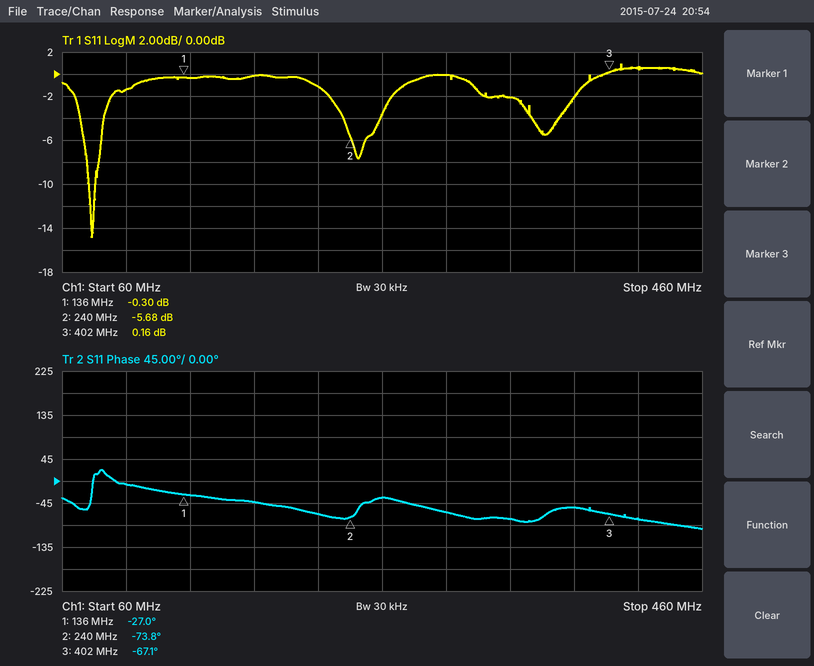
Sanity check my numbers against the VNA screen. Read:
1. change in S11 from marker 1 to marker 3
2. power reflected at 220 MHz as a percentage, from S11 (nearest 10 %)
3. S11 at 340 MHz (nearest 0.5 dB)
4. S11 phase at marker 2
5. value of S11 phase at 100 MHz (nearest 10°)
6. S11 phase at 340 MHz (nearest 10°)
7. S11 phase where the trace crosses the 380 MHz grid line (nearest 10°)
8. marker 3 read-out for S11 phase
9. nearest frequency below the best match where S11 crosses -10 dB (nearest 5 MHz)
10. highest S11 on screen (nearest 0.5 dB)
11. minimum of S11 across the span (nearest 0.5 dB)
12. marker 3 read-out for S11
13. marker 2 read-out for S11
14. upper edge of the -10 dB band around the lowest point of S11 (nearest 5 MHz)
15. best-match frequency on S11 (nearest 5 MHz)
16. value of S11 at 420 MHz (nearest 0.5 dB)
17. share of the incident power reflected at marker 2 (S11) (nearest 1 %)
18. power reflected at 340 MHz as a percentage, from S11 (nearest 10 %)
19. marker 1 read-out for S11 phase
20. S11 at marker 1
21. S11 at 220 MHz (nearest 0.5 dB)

0.46 dB
80 %
-2.0 dB
-73.8°
-10°
-80°
-50°
-67.1°
75 MHz
1.0 dB
-15.0 dB
0.16 dB
-5.68 dB
80 MHz
80 MHz
0.5 dB
27 %
60 %
-27.0°
-0.30 dB
-1.0 dB
